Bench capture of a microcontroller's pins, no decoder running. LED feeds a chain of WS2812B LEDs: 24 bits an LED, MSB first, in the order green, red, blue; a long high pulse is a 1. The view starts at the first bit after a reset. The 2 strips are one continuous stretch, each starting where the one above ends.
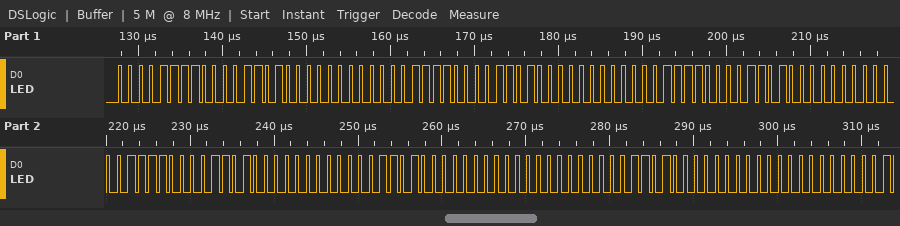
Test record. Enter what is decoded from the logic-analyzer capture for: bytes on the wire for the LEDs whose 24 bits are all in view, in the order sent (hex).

0F 0D 00 0F 0D 00 0F 0D 00 0F 0D 00 0D 00 00 0D 00 00
